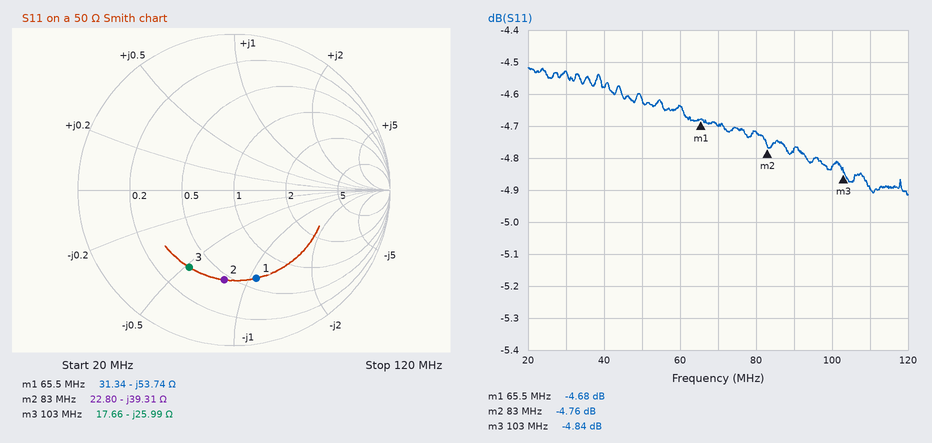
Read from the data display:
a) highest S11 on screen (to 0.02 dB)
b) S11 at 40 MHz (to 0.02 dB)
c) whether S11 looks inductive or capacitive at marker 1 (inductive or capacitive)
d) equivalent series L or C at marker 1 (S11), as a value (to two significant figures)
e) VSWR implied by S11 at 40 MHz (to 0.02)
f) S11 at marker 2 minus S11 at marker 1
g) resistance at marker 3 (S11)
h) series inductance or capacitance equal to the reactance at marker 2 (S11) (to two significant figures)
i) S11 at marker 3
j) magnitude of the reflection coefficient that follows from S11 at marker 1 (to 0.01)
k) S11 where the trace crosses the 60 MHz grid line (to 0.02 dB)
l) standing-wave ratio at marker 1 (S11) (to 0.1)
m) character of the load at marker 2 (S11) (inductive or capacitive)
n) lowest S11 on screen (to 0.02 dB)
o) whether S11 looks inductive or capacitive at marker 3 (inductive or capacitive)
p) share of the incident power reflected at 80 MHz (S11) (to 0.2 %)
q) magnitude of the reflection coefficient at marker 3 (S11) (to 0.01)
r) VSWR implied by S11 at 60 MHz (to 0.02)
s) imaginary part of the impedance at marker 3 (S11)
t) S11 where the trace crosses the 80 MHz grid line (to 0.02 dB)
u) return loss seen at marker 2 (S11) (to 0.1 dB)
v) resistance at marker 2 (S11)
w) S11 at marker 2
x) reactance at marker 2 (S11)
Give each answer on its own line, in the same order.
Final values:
-4.52 dB
-4.58 dB
capacitive
45 pF
3.88
-0.08 dB
17.66 Ω
49 pF
-4.84 dB
0.58
-4.64 dB
3.8
capacitive
-4.92 dB
capacitive
33.8 %
0.57
3.84
-25.99 Ω
-4.72 dB
4.8 dB
22.80 Ω
-4.76 dB
-39.31 Ω
